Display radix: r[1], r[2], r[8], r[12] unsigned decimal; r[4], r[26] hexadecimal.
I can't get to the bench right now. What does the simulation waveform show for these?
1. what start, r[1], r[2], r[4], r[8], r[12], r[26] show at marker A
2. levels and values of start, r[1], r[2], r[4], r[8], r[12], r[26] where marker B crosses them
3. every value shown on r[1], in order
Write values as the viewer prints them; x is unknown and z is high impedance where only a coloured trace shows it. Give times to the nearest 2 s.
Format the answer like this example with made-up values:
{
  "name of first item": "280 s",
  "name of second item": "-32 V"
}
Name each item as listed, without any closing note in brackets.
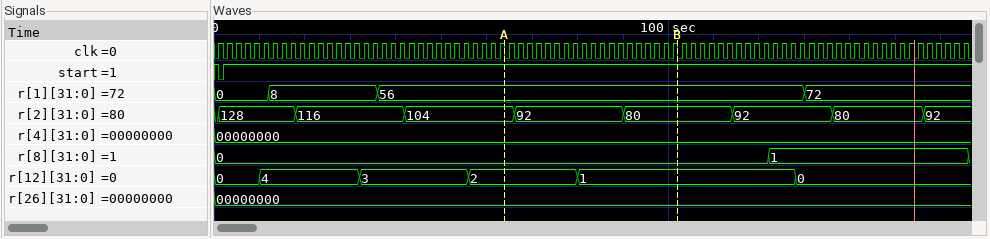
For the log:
{
  "what start, r[1], r[2], r[4], r[8], r[12], r[26] show at marker A": "start=1, r[1]=56, r[2]=104, r[4]=00000000, r[8]=0, r[12]=2, r[26]=00000000",
  "levels and values of start, r[1], r[2], r[4], r[8], r[12], r[26] where marker B crosses them": "start=1, r[1]=56, r[2]=80, r[4]=00000000, r[8]=0, r[12]=1, r[26]=00000000",
  "every value shown on r[1], in order": "0, 8, 56, 72"
}
